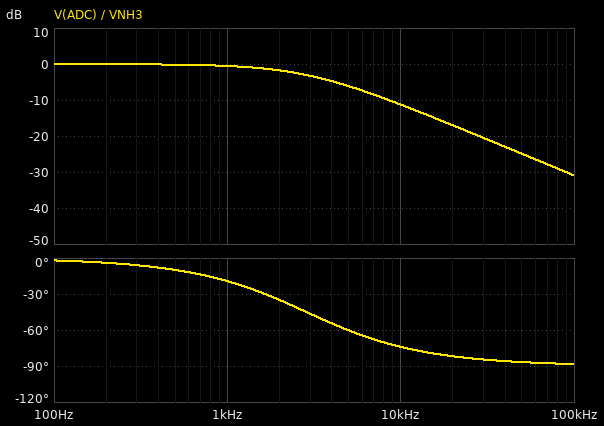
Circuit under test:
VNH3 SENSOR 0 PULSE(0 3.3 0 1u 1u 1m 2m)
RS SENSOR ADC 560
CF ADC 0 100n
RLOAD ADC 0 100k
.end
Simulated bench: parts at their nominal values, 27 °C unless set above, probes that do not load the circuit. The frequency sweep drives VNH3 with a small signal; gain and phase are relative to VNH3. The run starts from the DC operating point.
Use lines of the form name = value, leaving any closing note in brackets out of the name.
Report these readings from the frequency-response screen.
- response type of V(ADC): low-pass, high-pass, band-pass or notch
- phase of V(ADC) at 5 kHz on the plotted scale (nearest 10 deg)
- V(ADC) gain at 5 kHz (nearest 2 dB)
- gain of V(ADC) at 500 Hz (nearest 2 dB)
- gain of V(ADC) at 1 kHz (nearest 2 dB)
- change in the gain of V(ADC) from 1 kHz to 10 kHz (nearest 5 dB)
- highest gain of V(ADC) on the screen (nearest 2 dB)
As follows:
response type of V(ADC): low-pass, high-pass, band-pass or notch = low-pass
phase of V(ADC) at 5 kHz on the plotted scale = -60 deg
V(ADC) gain at 5 kHz = -6 dB
gain of V(ADC) at 500 Hz = 0 dB
gain of V(ADC) at 1 kHz = 0 dB
change in the gain of V(ADC) from 1 kHz to 10 kHz = -10 dB
highest gain of V(ADC) on the screen = 0 dB
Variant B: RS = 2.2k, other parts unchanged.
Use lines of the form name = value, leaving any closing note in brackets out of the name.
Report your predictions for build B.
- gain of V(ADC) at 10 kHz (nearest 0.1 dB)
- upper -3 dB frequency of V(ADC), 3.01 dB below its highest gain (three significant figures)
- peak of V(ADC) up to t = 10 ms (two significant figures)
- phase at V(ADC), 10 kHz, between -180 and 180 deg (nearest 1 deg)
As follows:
gain of V(ADC) at 10 kHz = -22.8 dB
upper -3 dB frequency of V(ADC), 3.01 dB below its highest gain = 739 Hz
peak of V(ADC) up to t = 10 ms = 3.2 V
phase at V(ADC), 10 kHz, between -180 and 180 deg = -86 deg
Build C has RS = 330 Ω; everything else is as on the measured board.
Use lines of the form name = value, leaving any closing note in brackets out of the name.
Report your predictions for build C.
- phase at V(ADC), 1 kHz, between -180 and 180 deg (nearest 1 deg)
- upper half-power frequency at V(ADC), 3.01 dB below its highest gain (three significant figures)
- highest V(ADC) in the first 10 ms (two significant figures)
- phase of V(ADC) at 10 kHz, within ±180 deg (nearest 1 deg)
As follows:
phase at V(ADC), 1 kHz, between -180 and 180 deg = -12 deg
upper half-power frequency at V(ADC), 3.01 dB below its highest gain = 4.84 kHz
highest V(ADC) in the first 10 ms = 3.3 V
phase of V(ADC) at 10 kHz, within ±180 deg = -64 deg
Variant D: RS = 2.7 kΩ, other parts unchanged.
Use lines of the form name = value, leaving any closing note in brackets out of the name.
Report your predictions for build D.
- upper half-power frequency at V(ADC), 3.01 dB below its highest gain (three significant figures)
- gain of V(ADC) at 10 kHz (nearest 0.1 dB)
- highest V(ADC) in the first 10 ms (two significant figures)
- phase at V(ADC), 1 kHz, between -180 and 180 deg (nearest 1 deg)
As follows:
upper half-power frequency at V(ADC), 3.01 dB below its highest gain = 605 Hz
gain of V(ADC) at 10 kHz = -24.6 dB
highest V(ADC) in the first 10 ms = 3.1 V
phase at V(ADC), 1 kHz, between -180 and 180 deg = -59 deg
